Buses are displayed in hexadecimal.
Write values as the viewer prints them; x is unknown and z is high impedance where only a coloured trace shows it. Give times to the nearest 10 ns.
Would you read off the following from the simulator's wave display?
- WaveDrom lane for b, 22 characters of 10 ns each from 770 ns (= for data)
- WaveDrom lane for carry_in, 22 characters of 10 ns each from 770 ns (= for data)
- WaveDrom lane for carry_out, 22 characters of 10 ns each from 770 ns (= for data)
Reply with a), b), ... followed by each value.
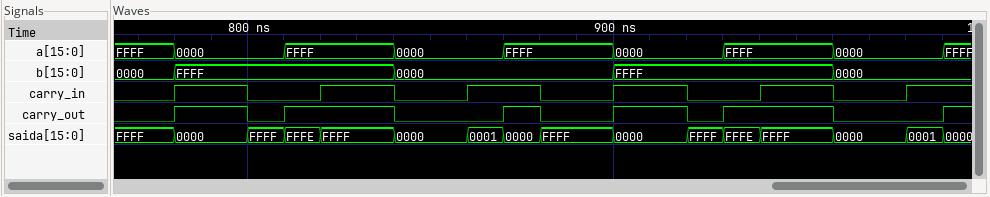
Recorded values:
a) {name: 'b', wave: '==.....=.....=.....=..', data: '0000 FFFF 0000 FFFF 0000'}
b) {name: 'carry_in', wave: '01.0.1.0.1.0.1.0.1.0.1'}
c) {name: 'carry_out', wave: '01.01..0..10.1.01..0..'}
